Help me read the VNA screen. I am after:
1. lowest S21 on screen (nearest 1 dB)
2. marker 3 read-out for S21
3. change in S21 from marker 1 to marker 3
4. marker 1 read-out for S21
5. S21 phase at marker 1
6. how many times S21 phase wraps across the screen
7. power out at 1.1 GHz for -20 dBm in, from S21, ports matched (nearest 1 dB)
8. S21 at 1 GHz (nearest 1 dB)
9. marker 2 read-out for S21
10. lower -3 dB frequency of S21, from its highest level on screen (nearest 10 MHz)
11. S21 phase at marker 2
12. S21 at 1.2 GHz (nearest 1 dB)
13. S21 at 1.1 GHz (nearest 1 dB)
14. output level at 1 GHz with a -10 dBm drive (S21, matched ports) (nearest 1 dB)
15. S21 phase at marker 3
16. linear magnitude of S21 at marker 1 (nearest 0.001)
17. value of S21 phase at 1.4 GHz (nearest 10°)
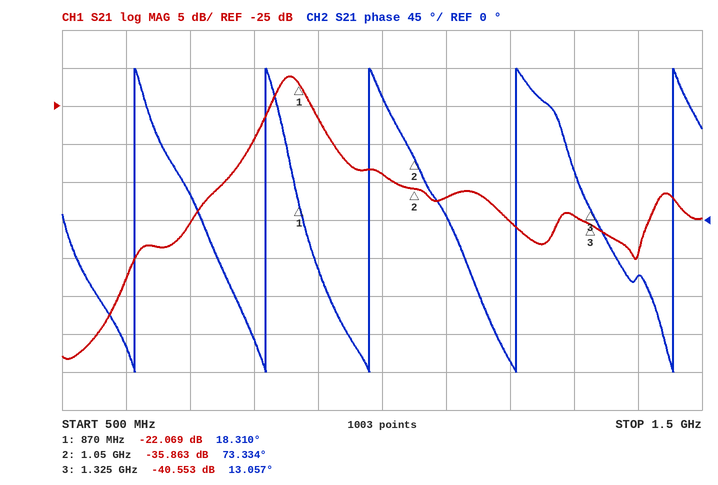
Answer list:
-58 dB
-40.553 dB
-18.484 dB
-22.069 dB
18.310°
5
-57 dBm
-34 dB
-35.863 dB
830 MHz
73.334°
-40 dB
-37 dB
-44 dBm
13.057°
0.079
-70°
